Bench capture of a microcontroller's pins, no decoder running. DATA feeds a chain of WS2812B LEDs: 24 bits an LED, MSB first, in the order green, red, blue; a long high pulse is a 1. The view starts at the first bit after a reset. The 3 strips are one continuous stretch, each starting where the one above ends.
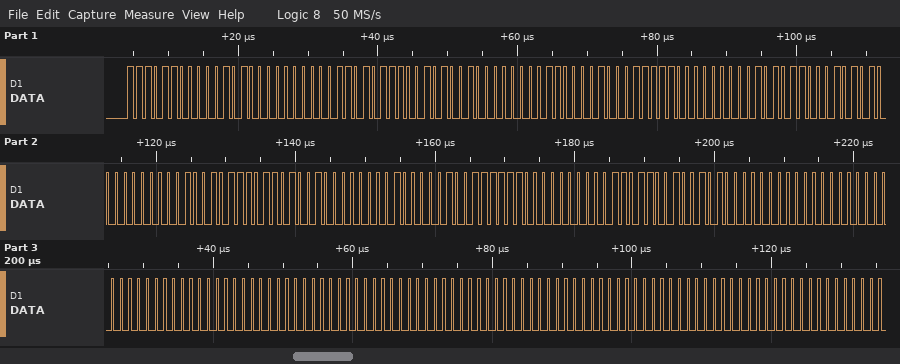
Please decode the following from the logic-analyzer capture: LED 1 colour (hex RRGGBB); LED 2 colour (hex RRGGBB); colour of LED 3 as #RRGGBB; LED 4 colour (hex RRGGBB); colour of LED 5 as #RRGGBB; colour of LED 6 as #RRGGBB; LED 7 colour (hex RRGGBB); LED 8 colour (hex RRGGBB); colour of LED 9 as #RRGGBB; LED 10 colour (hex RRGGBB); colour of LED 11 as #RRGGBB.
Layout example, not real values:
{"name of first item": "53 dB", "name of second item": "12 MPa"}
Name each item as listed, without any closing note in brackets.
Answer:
{"LED 1 colour": "#14EC00", "LED 2 colour": "#29D700", "colour of LED 3 as #RRGGBB": "#3EC200", "LED 4 colour": "#54AC00", "colour of LED 5 as #RRGGBB": "#699700", "colour of LED 6 as #RRGGBB": "#7E8200", "LED 7 colour": "#946C00", "LED 8 colour": "#000000", "colour of LED 9 as #RRGGBB": "#000000", "LED 10 colour": "#000000", "colour of LED 11 as #RRGGBB": "#000000"}
